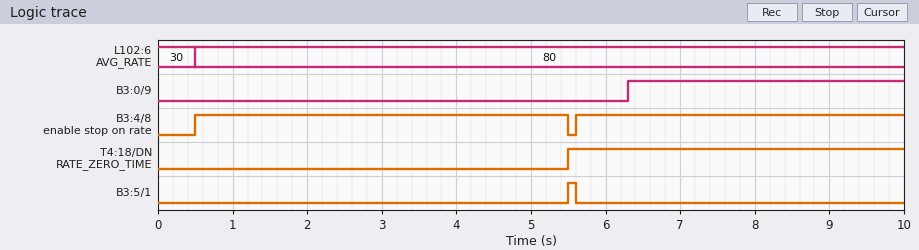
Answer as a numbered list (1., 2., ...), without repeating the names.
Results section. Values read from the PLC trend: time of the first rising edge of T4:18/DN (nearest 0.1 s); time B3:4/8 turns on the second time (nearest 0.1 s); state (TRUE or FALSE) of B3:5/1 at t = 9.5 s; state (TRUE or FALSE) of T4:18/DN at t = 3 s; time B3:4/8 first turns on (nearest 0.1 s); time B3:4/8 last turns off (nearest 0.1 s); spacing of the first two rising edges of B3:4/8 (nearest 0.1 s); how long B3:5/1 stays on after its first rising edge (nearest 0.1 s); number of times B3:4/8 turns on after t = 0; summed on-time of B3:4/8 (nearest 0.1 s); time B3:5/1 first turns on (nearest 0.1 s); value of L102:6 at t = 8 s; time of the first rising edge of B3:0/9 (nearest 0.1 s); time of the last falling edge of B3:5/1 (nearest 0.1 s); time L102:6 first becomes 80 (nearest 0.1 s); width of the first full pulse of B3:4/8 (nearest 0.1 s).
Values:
1. 5.5 s
2. 5.6 s
3. FALSE
4. FALSE
5. 0.5 s
6. 5.5 s
7. 5.1 s
8. 0.1 s
9. 2
10. 9.4 s
11. 5.5 s
12. 80
13. 6.3 s
14. 5.6 s
15. 0.5 s
16. 5.0 s
